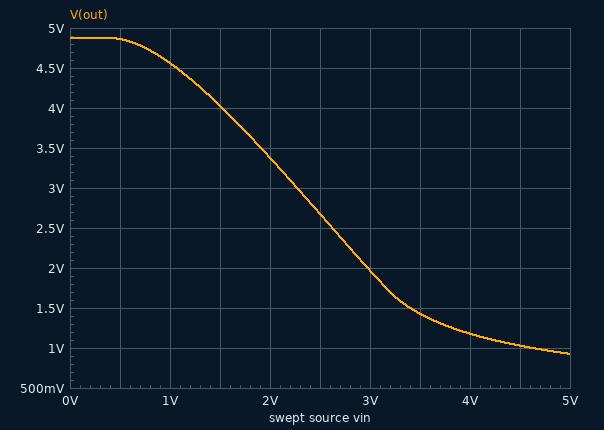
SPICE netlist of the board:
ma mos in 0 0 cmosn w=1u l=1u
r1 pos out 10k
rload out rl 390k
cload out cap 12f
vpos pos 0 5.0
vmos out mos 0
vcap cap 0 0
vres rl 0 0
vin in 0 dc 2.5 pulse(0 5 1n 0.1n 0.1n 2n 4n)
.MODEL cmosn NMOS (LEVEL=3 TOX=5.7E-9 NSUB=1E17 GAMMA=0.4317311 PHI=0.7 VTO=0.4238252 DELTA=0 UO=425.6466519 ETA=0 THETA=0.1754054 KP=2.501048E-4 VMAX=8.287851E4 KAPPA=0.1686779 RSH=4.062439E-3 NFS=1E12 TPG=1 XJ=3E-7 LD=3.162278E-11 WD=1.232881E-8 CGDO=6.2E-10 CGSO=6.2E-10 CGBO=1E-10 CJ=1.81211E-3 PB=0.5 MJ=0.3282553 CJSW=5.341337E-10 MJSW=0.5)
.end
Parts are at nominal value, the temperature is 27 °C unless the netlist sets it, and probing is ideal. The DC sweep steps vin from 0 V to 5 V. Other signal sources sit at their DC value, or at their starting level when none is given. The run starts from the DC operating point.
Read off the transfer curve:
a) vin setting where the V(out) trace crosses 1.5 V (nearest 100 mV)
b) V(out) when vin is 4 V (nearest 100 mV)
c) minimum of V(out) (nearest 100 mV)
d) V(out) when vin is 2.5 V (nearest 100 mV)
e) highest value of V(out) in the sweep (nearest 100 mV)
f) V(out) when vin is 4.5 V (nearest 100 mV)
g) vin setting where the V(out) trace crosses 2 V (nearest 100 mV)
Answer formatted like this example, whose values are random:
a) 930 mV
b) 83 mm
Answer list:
a) 3.4 V
b) 1.2 V
c) 900 mV
d) 2.7 V
e) 4.9 V
f) 1.0 V
g) 3.0 V
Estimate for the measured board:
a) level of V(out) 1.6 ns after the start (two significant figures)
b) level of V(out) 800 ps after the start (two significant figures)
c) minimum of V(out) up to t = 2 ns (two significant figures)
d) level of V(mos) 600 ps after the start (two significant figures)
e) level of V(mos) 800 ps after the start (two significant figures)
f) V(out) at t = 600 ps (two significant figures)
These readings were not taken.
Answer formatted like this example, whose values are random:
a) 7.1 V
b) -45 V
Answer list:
a) 930 mV
b) 4.9 V
c) 930 mV
d) 4.9 V
e) 4.9 V
f) 4.9 V
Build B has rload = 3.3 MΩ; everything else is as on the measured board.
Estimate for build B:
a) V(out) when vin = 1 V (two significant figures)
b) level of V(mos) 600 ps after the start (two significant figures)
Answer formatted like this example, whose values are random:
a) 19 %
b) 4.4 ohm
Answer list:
a) 4.7 V
b) 5.0 V
